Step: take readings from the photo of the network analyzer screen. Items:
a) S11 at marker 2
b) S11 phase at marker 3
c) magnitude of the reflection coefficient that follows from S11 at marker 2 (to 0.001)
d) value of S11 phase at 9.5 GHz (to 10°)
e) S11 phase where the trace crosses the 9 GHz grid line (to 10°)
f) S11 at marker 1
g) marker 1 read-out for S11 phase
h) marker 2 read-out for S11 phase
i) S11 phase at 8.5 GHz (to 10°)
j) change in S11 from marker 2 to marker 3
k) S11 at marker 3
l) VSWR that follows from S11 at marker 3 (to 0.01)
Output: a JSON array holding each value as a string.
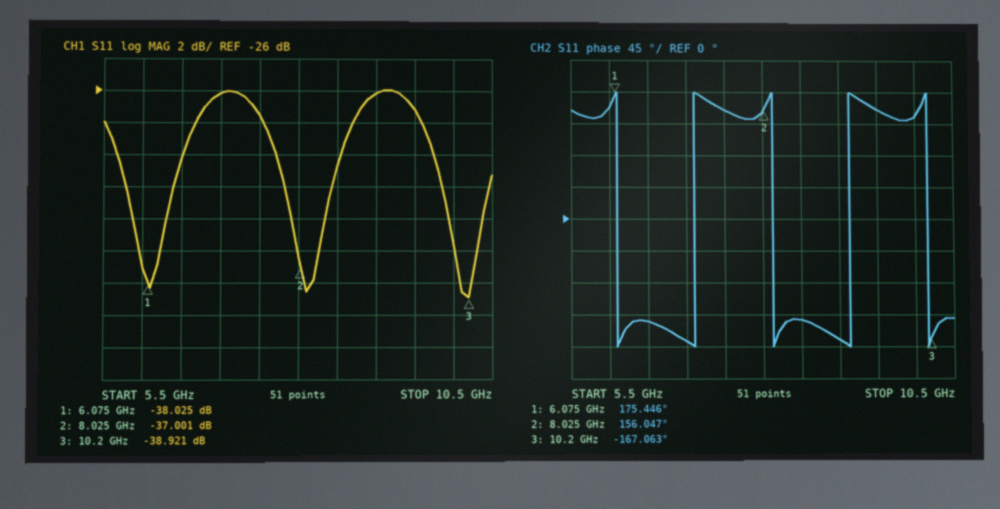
["-37.001 dB", "-167.063°", "0.014", "160°", "-170°", "-38.025 dB", "175.446°", "156.047°", "-140°", "-1.920 dB", "-38.921 dB", "1.02"]
